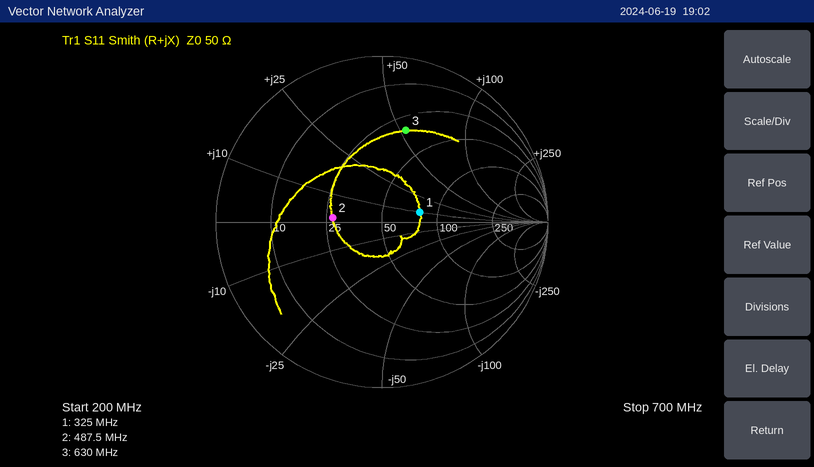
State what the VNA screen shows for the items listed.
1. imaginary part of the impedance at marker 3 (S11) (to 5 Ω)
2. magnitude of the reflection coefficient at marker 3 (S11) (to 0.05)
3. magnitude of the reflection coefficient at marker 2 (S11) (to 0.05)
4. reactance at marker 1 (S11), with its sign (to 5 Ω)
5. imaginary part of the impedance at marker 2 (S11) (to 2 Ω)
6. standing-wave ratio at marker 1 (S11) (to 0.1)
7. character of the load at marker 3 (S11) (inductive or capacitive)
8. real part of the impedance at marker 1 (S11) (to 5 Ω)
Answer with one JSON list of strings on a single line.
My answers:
["+55 Ω", "0.55", "0.30", "+10 Ω", "+2 Ω", "1.6", "inductive", "80 Ω"]
